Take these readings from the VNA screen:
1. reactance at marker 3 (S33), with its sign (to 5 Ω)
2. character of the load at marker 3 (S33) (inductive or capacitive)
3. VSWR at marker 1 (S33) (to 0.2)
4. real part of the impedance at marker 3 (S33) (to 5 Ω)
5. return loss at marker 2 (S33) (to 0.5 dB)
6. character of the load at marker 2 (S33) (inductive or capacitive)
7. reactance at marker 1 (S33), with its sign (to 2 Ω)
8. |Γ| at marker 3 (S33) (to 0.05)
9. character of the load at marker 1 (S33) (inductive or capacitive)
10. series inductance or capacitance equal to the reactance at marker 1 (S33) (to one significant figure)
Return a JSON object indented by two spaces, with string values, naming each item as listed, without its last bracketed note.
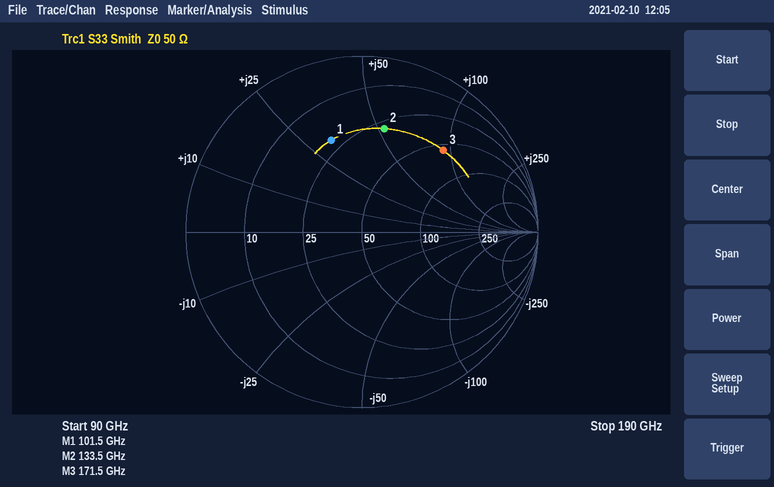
{
  "reactance at marker 3 (S33), with its sign": "+90 Ω",
  "character of the load at marker 3 (S33)": "inductive",
  "VSWR at marker 1 (S33)": "3.4",
  "real part of the impedance at marker 3 (S33)": "55 Ω",
  "return loss at marker 2 (S33)": "4.5 dB",
  "character of the load at marker 2 (S33)": "inductive",
  "reactance at marker 1 (S33), with its sign": "+32 Ω",
  "|Γ| at marker 3 (S33)": "0.65",
  "character of the load at marker 1 (S33)": "inductive",
  "series inductance or capacitance equal to the reactance at marker 1 (S33)": "50 pH"
}
